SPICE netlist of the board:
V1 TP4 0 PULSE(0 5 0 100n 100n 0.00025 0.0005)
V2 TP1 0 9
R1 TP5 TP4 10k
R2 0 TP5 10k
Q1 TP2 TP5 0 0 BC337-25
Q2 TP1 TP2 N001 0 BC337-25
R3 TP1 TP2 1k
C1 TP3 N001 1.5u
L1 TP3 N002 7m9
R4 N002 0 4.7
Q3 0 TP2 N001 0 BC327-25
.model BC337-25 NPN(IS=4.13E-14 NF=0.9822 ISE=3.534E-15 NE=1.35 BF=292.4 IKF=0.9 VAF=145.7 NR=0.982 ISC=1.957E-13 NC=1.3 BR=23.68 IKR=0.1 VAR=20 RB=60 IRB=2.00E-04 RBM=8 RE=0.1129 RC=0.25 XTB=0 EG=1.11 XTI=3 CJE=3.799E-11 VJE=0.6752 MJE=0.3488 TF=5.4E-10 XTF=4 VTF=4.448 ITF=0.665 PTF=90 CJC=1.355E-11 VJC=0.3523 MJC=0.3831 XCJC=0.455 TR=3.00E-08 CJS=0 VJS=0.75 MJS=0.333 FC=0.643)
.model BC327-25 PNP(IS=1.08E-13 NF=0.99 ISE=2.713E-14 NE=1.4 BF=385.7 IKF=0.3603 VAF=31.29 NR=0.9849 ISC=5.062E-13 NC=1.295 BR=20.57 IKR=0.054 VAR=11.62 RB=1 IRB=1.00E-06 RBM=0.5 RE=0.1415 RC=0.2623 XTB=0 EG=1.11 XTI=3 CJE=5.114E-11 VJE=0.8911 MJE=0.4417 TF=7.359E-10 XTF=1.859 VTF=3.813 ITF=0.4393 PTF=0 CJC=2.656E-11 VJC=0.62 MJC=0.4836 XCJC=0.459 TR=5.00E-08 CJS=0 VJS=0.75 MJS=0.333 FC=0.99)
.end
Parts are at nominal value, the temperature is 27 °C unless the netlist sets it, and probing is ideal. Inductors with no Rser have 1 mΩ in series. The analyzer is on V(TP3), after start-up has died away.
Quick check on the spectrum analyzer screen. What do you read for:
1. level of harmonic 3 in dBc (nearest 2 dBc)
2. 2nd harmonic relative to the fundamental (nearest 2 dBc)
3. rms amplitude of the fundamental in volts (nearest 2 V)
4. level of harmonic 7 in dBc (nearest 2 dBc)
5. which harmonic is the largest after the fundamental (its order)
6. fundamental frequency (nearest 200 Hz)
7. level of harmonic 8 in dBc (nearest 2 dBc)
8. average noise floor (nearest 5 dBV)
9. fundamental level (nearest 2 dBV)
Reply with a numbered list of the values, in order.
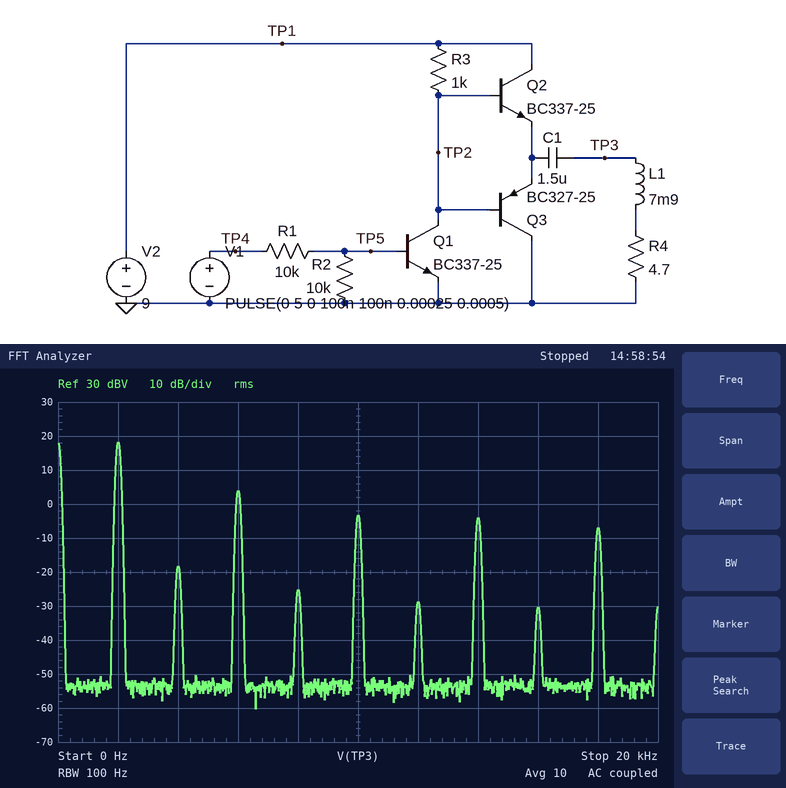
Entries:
1. -14 dBc
2. -36 dBc
3. 8 V
4. -22 dBc
5. 3
6. 2.0 kHz
7. -48 dBc
8. -55 dBV
9. 18 dBV
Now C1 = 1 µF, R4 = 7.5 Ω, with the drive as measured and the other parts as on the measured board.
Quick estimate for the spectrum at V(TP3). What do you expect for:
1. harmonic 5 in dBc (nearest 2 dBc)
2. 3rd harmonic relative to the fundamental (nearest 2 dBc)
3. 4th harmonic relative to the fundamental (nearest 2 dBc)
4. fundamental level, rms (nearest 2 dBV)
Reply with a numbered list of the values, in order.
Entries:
1. -26 dBc
2. -20 dBc
3. -46 dBc
4. 24 dBV
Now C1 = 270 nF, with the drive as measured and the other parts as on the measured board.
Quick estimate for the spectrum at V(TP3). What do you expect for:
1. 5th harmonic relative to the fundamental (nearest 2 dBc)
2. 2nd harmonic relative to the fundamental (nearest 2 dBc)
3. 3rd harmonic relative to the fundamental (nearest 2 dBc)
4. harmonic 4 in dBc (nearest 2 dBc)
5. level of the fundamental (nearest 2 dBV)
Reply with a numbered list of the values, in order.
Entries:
1. -8 dBc
2. -22 dBc
3. 0 dBc
4. -44 dBc
5. 6 dBV
